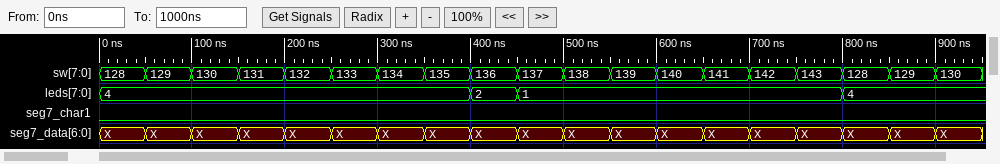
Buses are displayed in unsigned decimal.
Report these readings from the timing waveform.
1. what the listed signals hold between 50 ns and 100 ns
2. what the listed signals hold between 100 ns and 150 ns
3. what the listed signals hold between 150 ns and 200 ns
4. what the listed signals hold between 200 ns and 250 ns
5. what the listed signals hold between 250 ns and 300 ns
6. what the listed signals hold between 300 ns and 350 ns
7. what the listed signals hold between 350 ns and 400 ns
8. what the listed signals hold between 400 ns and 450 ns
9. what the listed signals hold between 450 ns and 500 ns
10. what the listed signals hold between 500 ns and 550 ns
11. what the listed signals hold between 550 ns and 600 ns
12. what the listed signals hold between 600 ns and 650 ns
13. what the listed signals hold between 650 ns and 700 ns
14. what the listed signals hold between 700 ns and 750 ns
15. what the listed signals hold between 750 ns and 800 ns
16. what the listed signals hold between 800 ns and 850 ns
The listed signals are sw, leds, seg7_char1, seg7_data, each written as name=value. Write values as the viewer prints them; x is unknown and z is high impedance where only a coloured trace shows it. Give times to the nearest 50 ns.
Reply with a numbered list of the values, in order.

1. sw=129, leds=4, seg7_char1=0, seg7_data=X
2. sw=130, leds=4, seg7_char1=0, seg7_data=X
3. sw=131, leds=4, seg7_char1=0, seg7_data=X
4. sw=132, leds=4, seg7_char1=0, seg7_data=X
5. sw=133, leds=4, seg7_char1=0, seg7_data=X
6. sw=134, leds=4, seg7_char1=0, seg7_data=X
7. sw=135, leds=4, seg7_char1=0, seg7_data=X
8. sw=136, leds=2, seg7_char1=0, seg7_data=X
9. sw=137, leds=1, seg7_char1=0, seg7_data=X
10. sw=138, leds=1, seg7_char1=0, seg7_data=X
11. sw=139, leds=1, seg7_char1=0, seg7_data=X
12. sw=140, leds=1, seg7_char1=0, seg7_data=X
13. sw=141, leds=1, seg7_char1=0, seg7_data=X
14. sw=142, leds=1, seg7_char1=0, seg7_data=X
15. sw=143, leds=1, seg7_char1=0, seg7_data=X
16. sw=128, leds=4, seg7_char1=0, seg7_data=X
